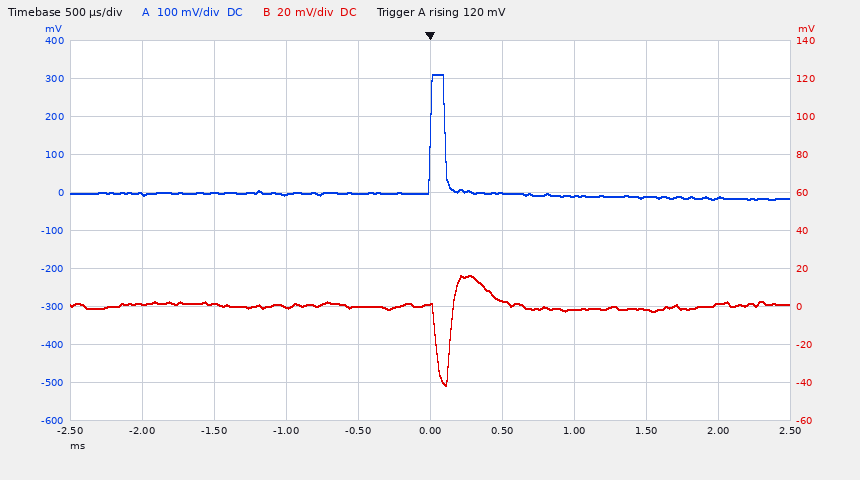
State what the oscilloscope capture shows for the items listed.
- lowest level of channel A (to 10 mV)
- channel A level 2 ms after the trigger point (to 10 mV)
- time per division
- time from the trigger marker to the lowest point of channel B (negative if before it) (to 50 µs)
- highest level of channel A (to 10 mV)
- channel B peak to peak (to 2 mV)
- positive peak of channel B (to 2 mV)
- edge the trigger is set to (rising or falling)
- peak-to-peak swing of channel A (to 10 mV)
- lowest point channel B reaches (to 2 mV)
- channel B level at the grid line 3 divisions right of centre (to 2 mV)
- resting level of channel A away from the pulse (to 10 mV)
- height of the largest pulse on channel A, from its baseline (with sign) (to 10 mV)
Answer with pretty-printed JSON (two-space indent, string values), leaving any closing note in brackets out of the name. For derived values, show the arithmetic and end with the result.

{
  "lowest level of channel A": "-20 mV",
  "channel A level 2 ms after the trigger point": "-10 mV",
  "time per division": "500 µs",
  "time from the trigger marker to the lowest point of channel B (negative if before it)": "+100 µs",
  "highest level of channel A": "310 mV",
  "channel B peak to peak": "16 mV − (-42 mV) = 58 mV",
  "positive peak of channel B": "16 mV",
  "edge the trigger is set to": "rising",
  "peak-to-peak swing of channel A": "310 mV − (-20 mV) = 330 mV",
  "lowest point channel B reaches": "-42 mV",
  "channel B level at the grid line 3 divisions right of centre": "-2 mV",
  "resting level of channel A away from the pulse": "0 mV",
  "height of the largest pulse on channel A, from its baseline (with sign)": "310 mV − (0 mV) = +310 mV"
}
